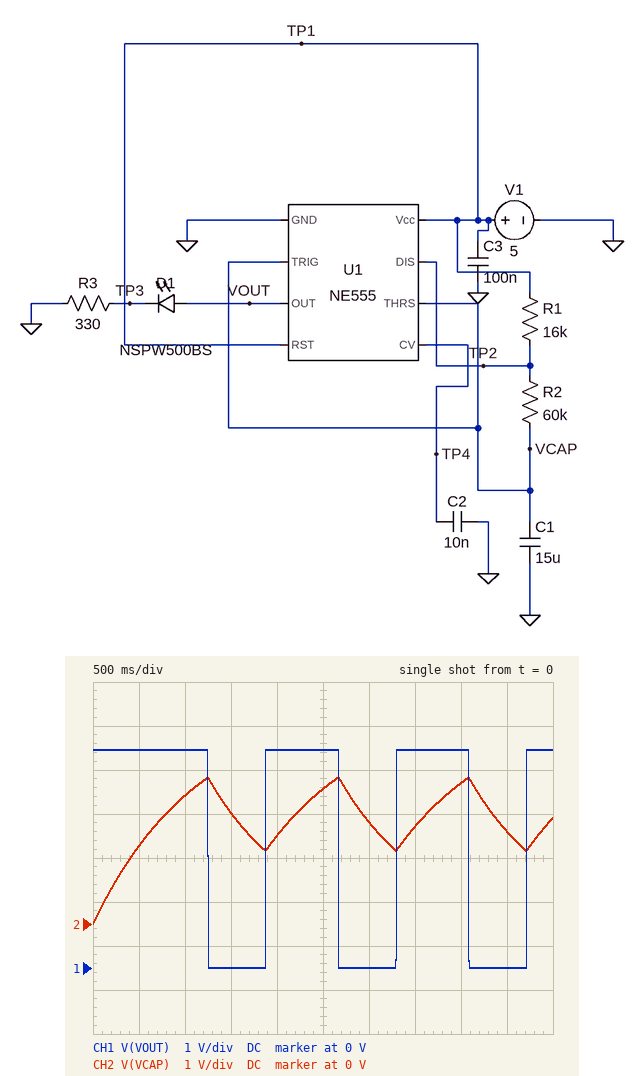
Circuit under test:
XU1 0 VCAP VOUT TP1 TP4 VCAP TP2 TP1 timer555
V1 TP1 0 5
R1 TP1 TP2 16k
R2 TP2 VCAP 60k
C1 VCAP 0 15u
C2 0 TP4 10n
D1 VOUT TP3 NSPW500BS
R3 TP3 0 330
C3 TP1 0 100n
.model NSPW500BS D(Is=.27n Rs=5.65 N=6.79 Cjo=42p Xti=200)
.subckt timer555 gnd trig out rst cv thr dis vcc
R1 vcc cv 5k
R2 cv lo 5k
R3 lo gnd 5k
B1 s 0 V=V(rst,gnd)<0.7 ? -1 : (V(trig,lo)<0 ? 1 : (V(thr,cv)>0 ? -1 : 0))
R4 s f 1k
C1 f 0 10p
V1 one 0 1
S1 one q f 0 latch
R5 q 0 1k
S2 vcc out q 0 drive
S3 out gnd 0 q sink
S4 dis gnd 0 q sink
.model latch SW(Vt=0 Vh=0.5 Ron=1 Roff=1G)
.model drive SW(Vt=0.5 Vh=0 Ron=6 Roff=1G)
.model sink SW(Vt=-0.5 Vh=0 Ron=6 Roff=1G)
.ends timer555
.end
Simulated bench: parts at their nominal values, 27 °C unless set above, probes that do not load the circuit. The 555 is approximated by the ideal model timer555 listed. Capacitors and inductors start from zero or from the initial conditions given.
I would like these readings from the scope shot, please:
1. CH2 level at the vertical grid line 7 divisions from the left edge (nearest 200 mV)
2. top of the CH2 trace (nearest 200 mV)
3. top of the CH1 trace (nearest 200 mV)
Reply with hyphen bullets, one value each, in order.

- 2.2 V
- 3.4 V
- 5.0 V
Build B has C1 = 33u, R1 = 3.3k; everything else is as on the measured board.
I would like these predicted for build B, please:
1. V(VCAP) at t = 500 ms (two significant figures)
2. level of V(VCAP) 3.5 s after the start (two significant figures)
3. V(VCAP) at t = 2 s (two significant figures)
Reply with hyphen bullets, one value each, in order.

- 1.1 V
- 1.8 V
- 3.1 V
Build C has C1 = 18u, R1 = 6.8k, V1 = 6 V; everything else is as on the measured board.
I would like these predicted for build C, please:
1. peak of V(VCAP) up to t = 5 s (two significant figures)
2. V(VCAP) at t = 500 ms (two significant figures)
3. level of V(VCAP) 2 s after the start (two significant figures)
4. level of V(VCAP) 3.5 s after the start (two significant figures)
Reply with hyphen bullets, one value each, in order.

- 4.0 V
- 2.0 V
- 2.1 V
- 2.3 V
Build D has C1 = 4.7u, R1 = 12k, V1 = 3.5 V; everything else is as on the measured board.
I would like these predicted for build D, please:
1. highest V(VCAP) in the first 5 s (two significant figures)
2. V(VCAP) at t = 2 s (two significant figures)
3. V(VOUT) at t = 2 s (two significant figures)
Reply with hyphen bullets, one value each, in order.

- 2.3 V
- 2.0 V
- 3.5 V
